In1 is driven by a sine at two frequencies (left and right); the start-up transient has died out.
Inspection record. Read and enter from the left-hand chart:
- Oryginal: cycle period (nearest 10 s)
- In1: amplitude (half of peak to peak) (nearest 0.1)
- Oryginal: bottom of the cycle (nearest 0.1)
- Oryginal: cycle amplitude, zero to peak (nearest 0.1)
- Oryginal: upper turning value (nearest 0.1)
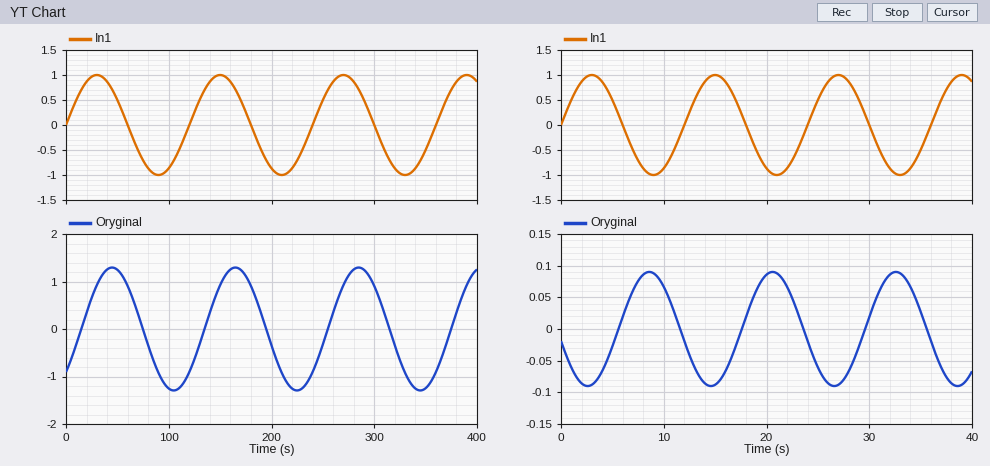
120 s
1.0
-1.3
1.3
1.3
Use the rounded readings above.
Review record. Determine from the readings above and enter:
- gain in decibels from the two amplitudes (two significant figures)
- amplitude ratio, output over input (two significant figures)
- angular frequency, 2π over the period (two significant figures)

2.3 dB
1.3
0.052 rad/s
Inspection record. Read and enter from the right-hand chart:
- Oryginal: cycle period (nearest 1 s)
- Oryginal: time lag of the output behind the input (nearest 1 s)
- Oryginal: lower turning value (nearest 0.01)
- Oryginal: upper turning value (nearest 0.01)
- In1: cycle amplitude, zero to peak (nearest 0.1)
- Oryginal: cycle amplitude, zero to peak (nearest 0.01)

12 s
6 s
-0.09
0.09
1.0
0.09
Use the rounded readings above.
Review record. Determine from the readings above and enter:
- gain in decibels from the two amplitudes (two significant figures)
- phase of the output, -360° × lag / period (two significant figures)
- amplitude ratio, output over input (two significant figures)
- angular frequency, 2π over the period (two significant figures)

-21 dB
-180°
0.090
0.52 rad/s
